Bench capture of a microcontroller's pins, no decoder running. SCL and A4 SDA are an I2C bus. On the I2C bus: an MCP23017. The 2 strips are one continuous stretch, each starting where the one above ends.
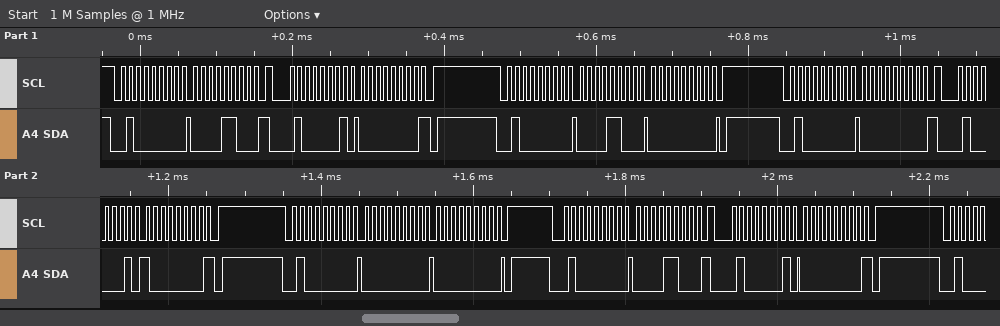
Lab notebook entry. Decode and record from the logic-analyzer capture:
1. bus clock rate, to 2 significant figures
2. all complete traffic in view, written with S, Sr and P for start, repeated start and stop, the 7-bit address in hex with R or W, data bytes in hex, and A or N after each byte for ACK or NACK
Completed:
100 kHz
S 20W A 0C A Sr 20R A 00 N P S 20W A 0C A 00 A P S 20W A 00 A Sr 20R A 80 N P S 20W A 00 A 00 A P S 20W A 0C A Sr 20R A 00 N P
